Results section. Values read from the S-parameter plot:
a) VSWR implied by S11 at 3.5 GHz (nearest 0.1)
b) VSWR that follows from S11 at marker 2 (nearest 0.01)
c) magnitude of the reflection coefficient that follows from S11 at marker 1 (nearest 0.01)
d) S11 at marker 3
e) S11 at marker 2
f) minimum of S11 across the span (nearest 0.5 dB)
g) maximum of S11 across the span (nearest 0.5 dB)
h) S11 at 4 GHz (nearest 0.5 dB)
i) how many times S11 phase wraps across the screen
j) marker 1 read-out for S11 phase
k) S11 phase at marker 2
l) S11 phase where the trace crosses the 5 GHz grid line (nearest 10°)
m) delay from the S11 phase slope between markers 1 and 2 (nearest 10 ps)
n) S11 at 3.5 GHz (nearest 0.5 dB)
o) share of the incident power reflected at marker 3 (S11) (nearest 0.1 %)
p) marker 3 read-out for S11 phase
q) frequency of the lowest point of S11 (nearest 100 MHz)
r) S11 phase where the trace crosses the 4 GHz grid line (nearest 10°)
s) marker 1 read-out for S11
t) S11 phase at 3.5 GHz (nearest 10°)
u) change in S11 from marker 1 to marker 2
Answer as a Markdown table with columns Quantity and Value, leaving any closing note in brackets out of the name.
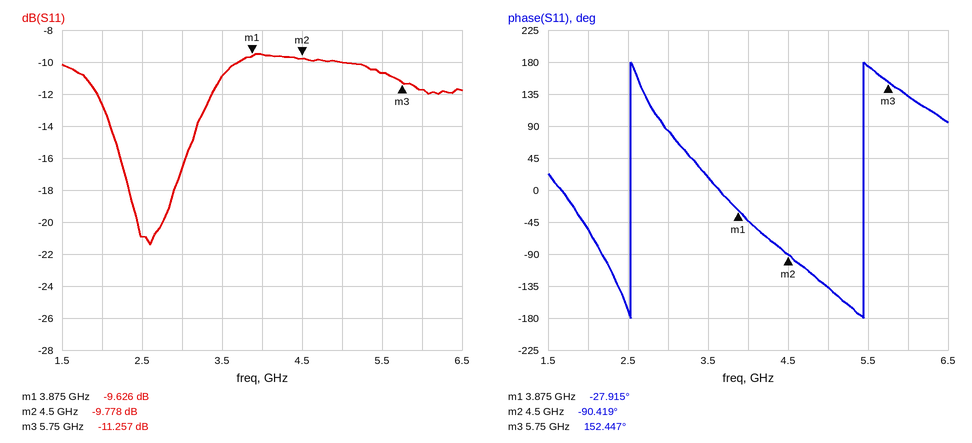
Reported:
| Quantity | Value |
|---|---|
| VSWR implied by S11 at 3.5 GHz | 1.8 |
| VSWR that follows from S11 at marker 2 | 1.96 |
| magnitude of the reflection coefficient that follows from S11 at marker 1 | 0.33 |
| S11 at marker 3 | -11.257 dB |
| S11 at marker 2 | -9.778 dB |
| minimum of S11 across the span | -21.5 dB |
| maximum of S11 across the span | -9.5 dB |
| S11 at 4 GHz | -9.5 dB |
| how many times S11 phase wraps across the screen | 2 |
| marker 1 read-out for S11 phase | -27.915° |
| S11 phase at marker 2 | -90.419° |
| S11 phase where the trace crosses the 5 GHz grid line | -140° |
| delay from the S11 phase slope between markers 1 and 2 | 280 ps |
| S11 at 3.5 GHz | -11.0 dB |
| share of the incident power reflected at marker 3 (S11) | 7.5 % |
| marker 3 read-out for S11 phase | 152.447° |
| frequency of the lowest point of S11 | 2.6 GHz |
| S11 phase where the trace crosses the 4 GHz grid line | -40° |
| marker 1 read-out for S11 | -9.626 dB |
| S11 phase at 3.5 GHz | 20° |
| change in S11 from marker 1 to marker 2 | -0.152 dB |
